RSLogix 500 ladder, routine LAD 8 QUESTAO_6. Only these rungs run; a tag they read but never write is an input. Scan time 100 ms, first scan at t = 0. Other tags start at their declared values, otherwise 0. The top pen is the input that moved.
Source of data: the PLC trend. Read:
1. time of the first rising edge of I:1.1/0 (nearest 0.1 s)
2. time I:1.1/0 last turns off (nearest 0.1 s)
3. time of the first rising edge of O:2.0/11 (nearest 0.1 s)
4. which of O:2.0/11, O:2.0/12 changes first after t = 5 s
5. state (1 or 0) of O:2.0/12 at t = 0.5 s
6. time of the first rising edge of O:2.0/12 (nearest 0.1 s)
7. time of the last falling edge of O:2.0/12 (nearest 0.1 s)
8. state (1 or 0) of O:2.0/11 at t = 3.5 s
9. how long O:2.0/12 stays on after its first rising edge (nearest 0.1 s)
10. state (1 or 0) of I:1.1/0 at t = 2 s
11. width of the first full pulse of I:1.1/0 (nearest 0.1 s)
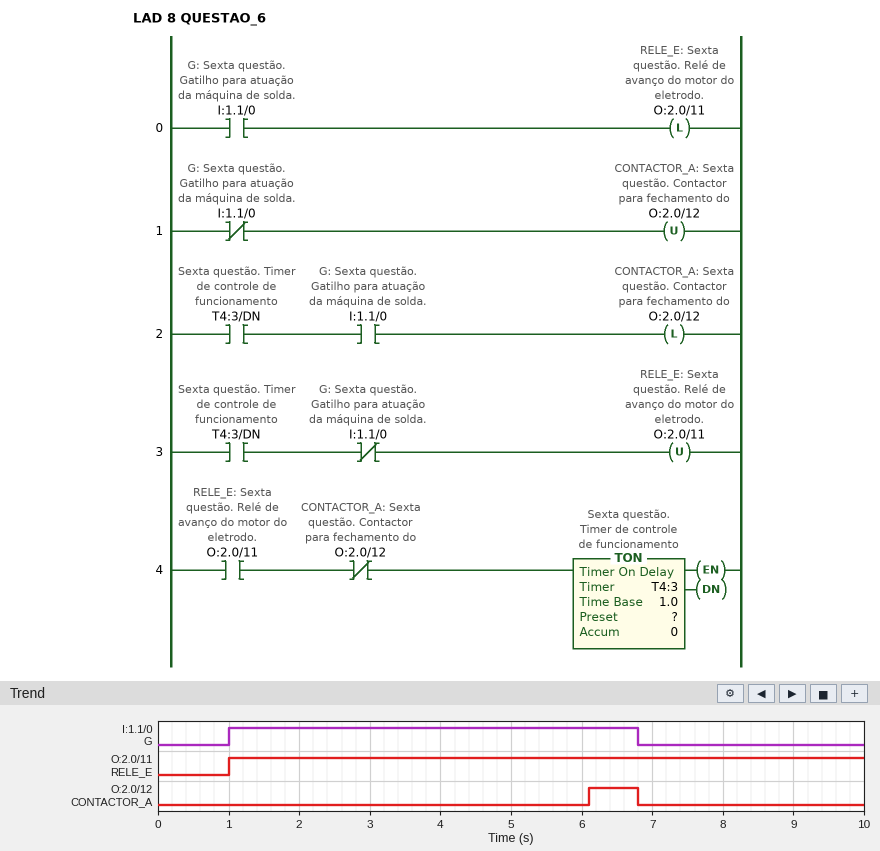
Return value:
1.0 s
6.8 s
1.0 s
O:2.0/12
0
6.1 s
6.8 s
1
0.7 s
1
5.8 s
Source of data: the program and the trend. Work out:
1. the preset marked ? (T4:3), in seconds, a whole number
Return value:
5 s
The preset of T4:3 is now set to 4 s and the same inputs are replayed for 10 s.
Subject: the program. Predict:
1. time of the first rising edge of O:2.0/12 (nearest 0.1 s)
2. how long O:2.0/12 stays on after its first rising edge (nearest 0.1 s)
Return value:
5.1 s
1.7 s
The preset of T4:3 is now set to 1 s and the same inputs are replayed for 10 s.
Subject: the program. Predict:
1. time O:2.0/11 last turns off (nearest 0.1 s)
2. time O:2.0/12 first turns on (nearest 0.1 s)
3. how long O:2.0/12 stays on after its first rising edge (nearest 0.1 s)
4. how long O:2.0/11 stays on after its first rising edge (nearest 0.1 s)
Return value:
7.9 s
2.1 s
4.7 s
6.9 s
